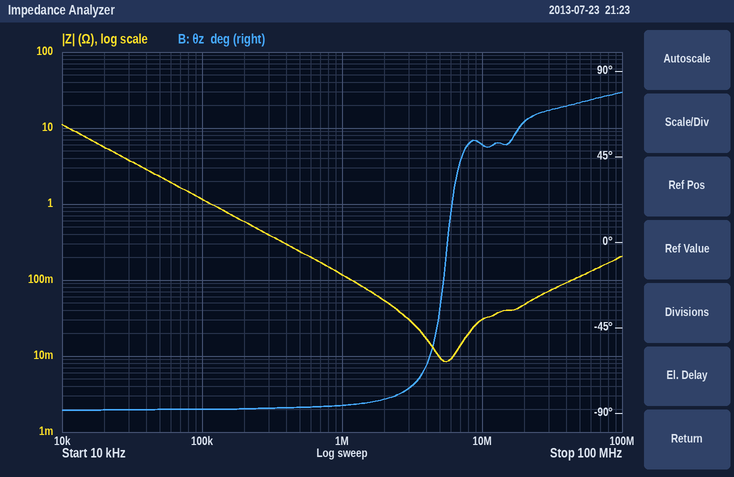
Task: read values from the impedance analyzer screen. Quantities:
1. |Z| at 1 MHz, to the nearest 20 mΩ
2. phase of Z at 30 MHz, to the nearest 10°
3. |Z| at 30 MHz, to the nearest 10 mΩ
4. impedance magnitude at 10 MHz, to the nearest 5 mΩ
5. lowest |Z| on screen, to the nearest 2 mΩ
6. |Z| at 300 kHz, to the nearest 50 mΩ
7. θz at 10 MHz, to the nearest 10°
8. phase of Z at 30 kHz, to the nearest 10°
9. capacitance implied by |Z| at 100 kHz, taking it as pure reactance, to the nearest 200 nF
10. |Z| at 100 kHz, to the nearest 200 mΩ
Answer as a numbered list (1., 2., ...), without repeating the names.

1. 120 mΩ
2. 70°
3. 70 mΩ
4. 30 mΩ
5. 8 mΩ
6. 400 mΩ
7. 50°
8. -90°
9. 1.4 µF
10. 1.2 Ω
